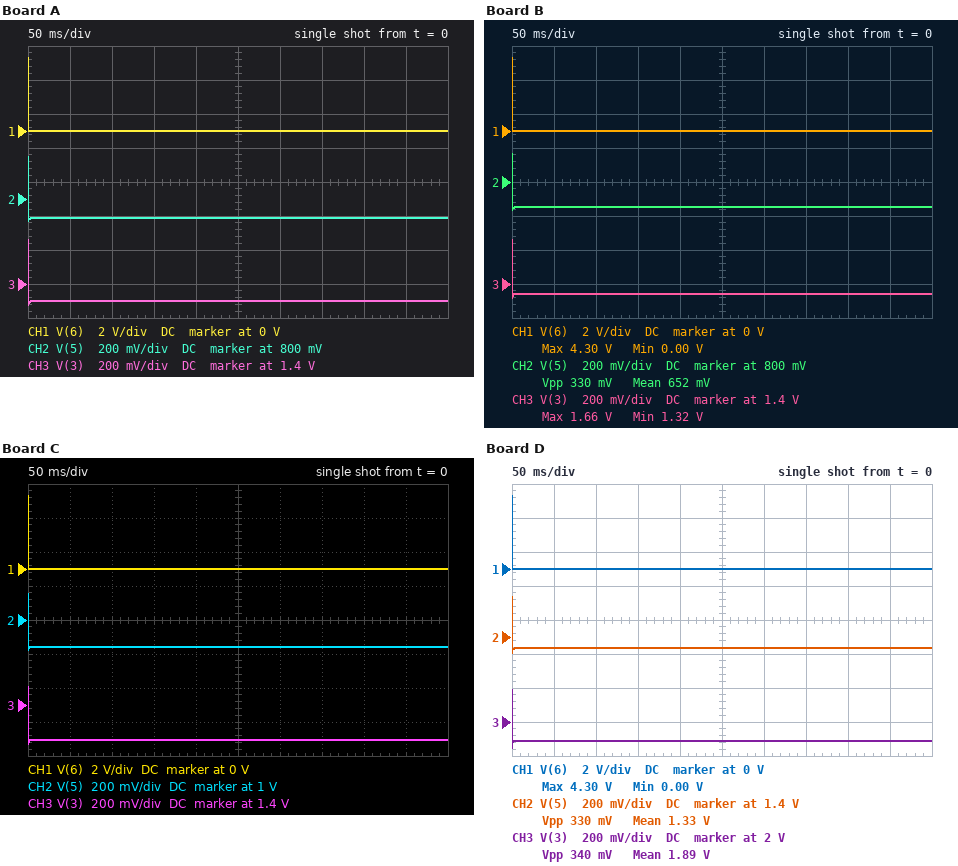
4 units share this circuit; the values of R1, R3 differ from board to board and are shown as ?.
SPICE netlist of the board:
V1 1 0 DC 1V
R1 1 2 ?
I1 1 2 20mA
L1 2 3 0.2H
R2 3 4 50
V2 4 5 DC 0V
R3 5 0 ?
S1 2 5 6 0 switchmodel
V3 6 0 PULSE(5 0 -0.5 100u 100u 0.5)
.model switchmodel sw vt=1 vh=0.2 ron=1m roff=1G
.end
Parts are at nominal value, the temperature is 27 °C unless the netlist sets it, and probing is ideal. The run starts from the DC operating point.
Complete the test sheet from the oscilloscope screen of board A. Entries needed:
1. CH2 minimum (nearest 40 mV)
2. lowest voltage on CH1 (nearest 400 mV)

680 mV
0 V
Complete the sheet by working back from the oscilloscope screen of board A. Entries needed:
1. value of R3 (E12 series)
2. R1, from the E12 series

56 Ω
39 Ω
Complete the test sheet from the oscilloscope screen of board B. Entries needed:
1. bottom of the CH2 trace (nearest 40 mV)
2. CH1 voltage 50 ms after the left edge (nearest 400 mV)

640 mV
0 V
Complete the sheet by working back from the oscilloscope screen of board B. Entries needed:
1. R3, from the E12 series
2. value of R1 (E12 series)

47 Ω
56 Ω
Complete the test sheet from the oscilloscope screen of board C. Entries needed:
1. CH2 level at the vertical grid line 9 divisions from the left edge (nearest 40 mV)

840 mV
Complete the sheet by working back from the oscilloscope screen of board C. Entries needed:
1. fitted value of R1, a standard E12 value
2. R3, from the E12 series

15 Ω
120 Ω
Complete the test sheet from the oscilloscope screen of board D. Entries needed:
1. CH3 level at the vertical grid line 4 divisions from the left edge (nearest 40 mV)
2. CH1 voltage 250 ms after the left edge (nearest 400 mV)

1.88 V
0 V
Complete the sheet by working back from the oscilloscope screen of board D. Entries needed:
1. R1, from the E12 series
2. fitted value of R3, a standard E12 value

100 Ω
120 Ω
